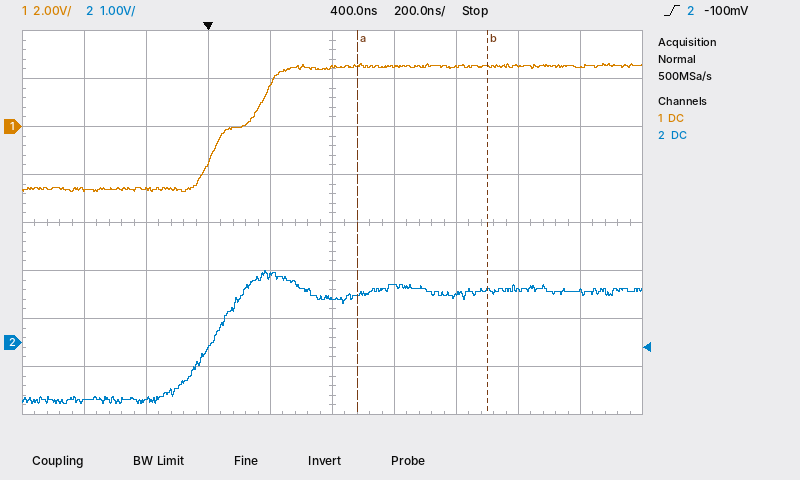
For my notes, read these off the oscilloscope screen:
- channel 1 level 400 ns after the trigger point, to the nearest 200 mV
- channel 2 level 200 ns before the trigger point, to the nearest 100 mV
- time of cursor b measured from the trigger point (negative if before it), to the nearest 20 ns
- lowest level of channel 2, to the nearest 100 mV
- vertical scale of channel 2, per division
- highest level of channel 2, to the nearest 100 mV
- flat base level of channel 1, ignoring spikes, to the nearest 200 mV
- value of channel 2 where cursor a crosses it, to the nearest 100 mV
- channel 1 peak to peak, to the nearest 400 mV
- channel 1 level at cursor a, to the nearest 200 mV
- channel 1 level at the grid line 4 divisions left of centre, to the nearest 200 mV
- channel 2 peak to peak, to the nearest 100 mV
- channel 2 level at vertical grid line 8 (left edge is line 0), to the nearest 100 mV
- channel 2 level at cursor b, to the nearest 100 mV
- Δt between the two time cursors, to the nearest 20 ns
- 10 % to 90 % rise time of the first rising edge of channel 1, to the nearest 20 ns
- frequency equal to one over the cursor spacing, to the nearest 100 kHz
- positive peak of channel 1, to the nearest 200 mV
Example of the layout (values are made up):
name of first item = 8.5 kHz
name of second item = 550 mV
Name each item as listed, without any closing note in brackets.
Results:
channel 1 level 400 ns after the trigger point, to the nearest 200 mV = 2.4 V
channel 2 level 200 ns before the trigger point, to the nearest 100 mV = -1.2 V
time of cursor b measured from the trigger point (negative if before it), to the nearest 20 ns = +900 ns
lowest level of channel 2, to the nearest 100 mV = -1.3 V
vertical scale of channel 2, per division = 1 V
highest level of channel 2, to the nearest 100 mV = 1.5 V
flat base level of channel 1, ignoring spikes, to the nearest 200 mV = -2.6 V
value of channel 2 where cursor a crosses it, to the nearest 100 mV = 1.0 V
channel 1 peak to peak, to the nearest 400 mV = 5.2 V
channel 1 level at cursor a, to the nearest 200 mV = 2.6 V
channel 1 level at the grid line 4 divisions left of centre, to the nearest 200 mV = -2.6 V
channel 2 peak to peak, to the nearest 100 mV = 2.8 V
channel 2 level at vertical grid line 8 (left edge is line 0), to the nearest 100 mV = 1.1 V
channel 2 level at cursor b, to the nearest 100 mV = 1.1 V
Δt between the two time cursors, to the nearest 20 ns = 420 ns
10 % to 90 % rise time of the first rising edge of channel 1, to the nearest 20 ns = 240 ns
frequency equal to one over the cursor spacing, to the nearest 100 kHz = 2.4 MHz
positive peak of channel 1, to the nearest 200 mV = 2.6 V
